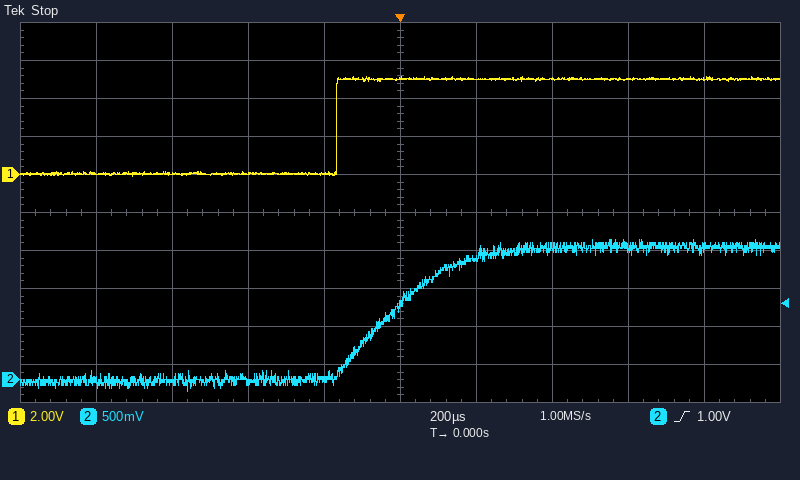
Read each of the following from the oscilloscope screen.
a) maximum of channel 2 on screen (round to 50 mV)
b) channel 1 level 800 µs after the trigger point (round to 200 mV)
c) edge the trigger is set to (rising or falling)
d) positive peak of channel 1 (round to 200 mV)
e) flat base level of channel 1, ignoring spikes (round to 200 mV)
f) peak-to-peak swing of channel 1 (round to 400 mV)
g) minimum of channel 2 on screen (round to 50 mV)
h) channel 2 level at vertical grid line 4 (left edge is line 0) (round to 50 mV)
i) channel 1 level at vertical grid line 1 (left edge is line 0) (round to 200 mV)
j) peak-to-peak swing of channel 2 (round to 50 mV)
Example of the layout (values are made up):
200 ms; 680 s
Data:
1.85 V; 5.0 V; rising; 5.2 V; 0.0 V; 5.2 V; -150 mV; 0 mV; 0.0 V; 2.00 V
